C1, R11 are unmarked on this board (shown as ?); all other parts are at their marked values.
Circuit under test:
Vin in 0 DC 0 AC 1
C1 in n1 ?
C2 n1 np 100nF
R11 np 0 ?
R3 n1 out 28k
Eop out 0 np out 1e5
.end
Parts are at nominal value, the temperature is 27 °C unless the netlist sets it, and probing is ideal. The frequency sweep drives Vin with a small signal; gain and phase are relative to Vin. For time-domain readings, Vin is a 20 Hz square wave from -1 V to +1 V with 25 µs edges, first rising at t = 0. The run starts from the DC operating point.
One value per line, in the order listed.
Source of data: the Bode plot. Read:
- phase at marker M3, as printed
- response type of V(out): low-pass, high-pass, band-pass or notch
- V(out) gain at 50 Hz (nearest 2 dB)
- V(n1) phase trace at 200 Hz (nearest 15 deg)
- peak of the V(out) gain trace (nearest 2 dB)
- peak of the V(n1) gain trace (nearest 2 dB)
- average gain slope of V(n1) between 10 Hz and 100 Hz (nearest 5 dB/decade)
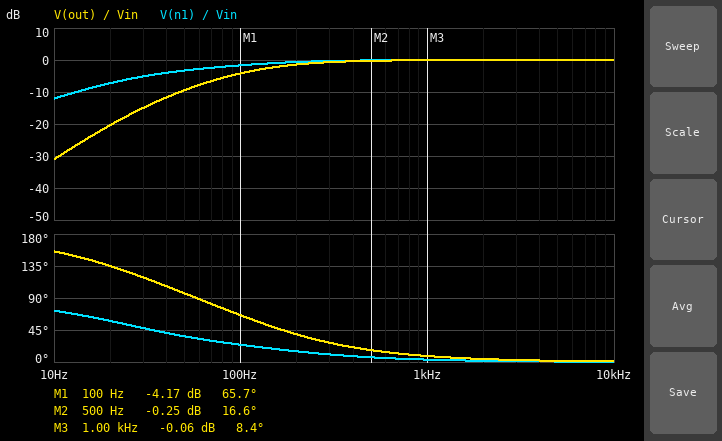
8.4 deg
high-pass
-10 dB
15 deg
0 dB
0 dB
10 dB/decade
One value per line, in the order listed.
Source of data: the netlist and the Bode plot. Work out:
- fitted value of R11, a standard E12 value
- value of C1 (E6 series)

18 kΩ
150 nF
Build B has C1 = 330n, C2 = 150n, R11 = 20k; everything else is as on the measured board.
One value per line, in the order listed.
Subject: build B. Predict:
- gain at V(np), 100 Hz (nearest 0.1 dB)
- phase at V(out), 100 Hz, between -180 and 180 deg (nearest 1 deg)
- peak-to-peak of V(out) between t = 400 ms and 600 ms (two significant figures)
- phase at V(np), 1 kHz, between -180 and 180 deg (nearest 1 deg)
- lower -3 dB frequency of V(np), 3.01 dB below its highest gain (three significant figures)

-1.5 dB
40 deg
4.1 V
4 deg
65.7 Hz
